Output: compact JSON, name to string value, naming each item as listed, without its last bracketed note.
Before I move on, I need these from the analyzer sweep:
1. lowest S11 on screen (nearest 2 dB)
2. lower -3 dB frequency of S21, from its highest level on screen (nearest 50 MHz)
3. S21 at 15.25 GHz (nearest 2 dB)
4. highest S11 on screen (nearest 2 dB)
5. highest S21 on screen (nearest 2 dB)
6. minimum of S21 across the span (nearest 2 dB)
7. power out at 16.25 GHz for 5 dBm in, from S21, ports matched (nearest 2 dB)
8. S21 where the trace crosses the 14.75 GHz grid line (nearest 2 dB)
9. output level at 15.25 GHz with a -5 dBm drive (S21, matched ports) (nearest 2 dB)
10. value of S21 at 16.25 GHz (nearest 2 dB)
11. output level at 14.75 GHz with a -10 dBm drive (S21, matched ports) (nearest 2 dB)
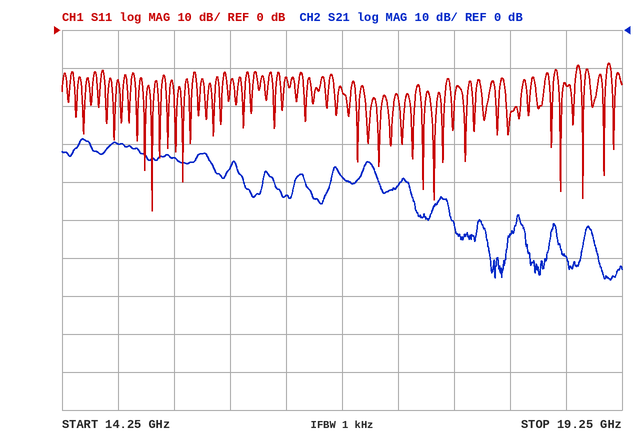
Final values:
{"lowest S11 on screen": "-48 dB", "lower -3 dB frequency of S21, from its highest level on screen": "14.35 GHz", "S21 at 15.25 GHz": "-34 dB", "highest S11 on screen": "-8 dB", "highest S21 on screen": "-28 dB", "minimum of S21 across the span": "-66 dB", "power out at 16.25 GHz for 5 dBm in, from S21, ports matched": "-38 dBm", "S21 where the trace crosses the 14.75 GHz grid line": "-30 dB", "output level at 15.25 GHz with a -5 dBm drive (S21, matched ports)": "-38 dBm", "value of S21 at 16.25 GHz": "-44 dB", "output level at 14.75 GHz with a -10 dBm drive (S21, matched ports)": "-40 dBm"}
